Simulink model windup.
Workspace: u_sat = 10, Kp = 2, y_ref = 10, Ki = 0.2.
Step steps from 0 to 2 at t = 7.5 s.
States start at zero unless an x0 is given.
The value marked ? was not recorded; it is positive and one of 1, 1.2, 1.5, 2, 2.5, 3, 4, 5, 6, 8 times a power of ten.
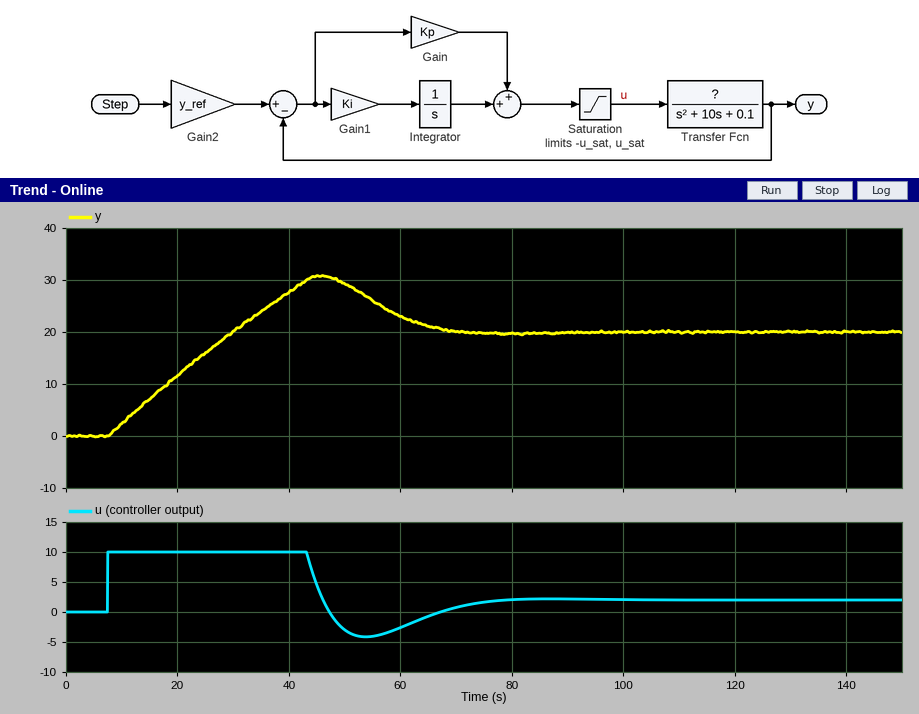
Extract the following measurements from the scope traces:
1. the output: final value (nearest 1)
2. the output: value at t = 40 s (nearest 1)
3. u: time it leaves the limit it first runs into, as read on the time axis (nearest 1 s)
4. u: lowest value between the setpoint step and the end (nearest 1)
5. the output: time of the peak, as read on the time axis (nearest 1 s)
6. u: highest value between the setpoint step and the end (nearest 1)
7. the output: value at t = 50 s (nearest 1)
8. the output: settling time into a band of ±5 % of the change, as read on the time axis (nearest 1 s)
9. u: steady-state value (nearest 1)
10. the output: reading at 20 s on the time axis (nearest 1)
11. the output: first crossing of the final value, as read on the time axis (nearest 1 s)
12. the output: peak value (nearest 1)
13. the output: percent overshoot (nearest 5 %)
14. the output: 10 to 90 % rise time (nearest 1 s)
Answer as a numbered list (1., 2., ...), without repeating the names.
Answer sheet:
1. 20
2. 28
3. 43 s
4. -4
5. 46 s
6. 10
7. 29
8. 65 s
9. 2
10. 12
11. 30 s
12. 31
13. 55 %
14. 18 s
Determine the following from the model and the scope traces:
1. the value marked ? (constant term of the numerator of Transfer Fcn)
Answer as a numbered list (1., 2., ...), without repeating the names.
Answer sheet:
1. 1
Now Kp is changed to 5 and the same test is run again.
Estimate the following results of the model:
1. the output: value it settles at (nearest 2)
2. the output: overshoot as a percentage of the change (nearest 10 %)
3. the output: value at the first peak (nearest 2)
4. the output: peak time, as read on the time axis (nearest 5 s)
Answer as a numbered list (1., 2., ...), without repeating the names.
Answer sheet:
1. 20
2. 30 %
3. 26
4. 40 s
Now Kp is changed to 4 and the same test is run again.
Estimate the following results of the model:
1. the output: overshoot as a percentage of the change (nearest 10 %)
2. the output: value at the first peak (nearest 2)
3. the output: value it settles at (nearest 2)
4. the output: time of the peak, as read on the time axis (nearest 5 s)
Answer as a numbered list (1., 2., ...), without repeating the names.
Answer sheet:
1. 40 %
2. 28
3. 20
4. 40 s
